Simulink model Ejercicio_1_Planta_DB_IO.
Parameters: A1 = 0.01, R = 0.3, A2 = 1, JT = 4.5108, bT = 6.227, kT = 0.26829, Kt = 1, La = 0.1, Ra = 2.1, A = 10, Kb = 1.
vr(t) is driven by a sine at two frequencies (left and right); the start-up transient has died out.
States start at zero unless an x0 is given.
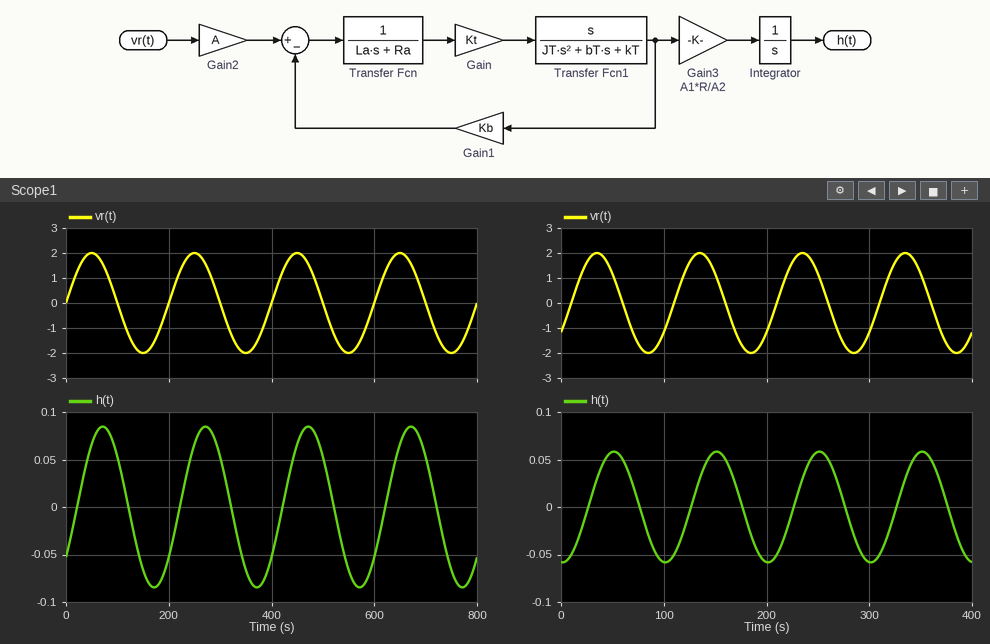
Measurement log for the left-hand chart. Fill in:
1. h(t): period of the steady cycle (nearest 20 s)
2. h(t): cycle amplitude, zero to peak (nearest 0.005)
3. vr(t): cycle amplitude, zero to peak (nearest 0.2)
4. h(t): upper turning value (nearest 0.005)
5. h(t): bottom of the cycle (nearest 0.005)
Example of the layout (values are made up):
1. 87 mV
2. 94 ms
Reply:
1. 200 s
2. 0.085
3. 2.0
4. 0.085
5. -0.085
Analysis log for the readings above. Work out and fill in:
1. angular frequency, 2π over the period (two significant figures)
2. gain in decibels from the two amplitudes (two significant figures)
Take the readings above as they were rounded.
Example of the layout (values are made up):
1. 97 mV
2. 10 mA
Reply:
1. 0.031 rad/s
2. -27 dB
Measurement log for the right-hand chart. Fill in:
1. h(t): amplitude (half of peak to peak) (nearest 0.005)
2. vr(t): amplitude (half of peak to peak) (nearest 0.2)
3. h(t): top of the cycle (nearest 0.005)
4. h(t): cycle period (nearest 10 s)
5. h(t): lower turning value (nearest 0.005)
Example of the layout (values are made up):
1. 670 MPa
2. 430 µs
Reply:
1. 0.060
2. 2.0
3. 0.060
4. 100 s
5. -0.060
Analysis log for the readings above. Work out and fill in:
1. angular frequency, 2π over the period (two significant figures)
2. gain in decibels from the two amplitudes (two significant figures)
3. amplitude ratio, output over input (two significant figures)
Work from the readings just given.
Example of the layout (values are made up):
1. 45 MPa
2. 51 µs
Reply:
1. 0.063 rad/s
2. -30 dB
3. 0.030
